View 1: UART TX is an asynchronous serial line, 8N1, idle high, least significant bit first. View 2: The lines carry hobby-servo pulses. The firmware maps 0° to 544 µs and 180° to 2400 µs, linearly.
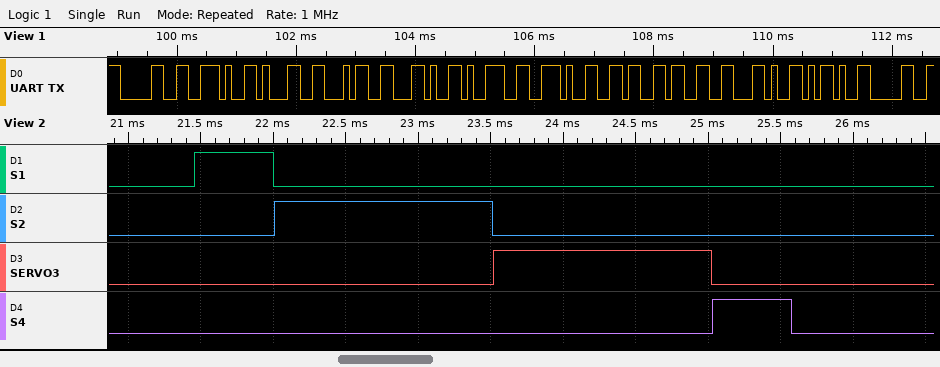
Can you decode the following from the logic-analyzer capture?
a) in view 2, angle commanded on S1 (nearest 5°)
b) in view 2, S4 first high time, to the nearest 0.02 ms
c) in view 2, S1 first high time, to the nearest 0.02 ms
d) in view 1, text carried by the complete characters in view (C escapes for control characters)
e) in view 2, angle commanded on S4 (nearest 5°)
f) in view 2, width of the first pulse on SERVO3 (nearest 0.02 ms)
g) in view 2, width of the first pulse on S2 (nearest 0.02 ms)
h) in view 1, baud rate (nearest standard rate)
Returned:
0°
0.54 ms
0.54 ms
"0.14,9.63,-0"
0°
1.50 ms
1.50 ms
9600 baud
